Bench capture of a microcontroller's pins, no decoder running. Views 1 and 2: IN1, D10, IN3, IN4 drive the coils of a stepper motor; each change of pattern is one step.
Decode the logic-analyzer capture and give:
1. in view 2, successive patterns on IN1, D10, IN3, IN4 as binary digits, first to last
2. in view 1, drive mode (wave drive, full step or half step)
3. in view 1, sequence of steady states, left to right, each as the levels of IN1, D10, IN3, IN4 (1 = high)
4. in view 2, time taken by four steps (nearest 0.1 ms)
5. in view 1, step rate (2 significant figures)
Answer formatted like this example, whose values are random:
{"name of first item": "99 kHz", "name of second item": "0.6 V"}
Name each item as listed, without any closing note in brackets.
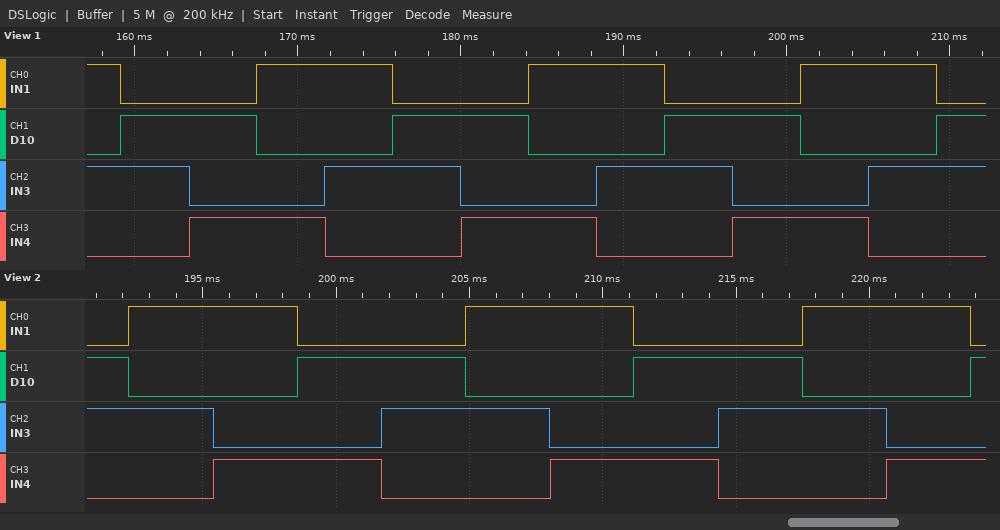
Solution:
{"in view 2, successive patterns on IN1, D10, IN3, IN4 as binary digits, first to last": "0110 1010 1001 0101 0110 1010 1001 0101 0110 1010 1001 0101", "in view 1, drive mode": "full step", "in view 1, sequence of steady states, left to right, each as the levels of IN1, D10, IN3, IN4": "1010 0110 0101 1001 1010 0110 0101 1001 1010 0110 0101 1001 1010 0110", "in view 2, time taken by four steps": "12.6 ms", "in view 1, step rate": "240 steps/s"}
